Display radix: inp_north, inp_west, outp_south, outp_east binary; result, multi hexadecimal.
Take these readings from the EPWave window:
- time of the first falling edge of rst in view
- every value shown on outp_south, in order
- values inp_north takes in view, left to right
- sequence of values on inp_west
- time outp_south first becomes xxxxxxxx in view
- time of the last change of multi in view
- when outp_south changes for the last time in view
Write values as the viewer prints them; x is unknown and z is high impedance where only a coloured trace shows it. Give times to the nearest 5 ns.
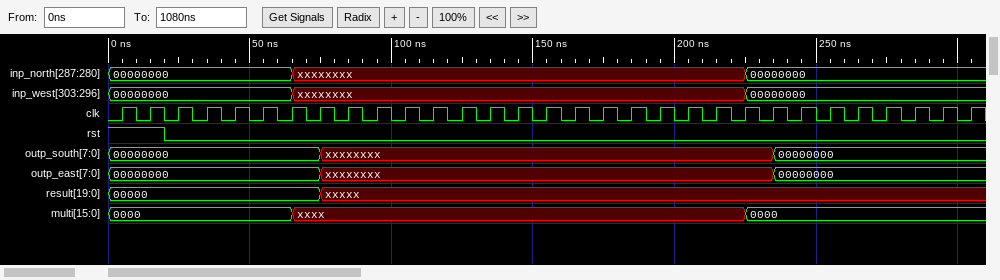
20 ns
00000000, xxxxxxxx, 00000000
00000000, xxxxxxxx, 00000000
00000000, xxxxxxxx, 00000000
75 ns
225 ns
235 ns
